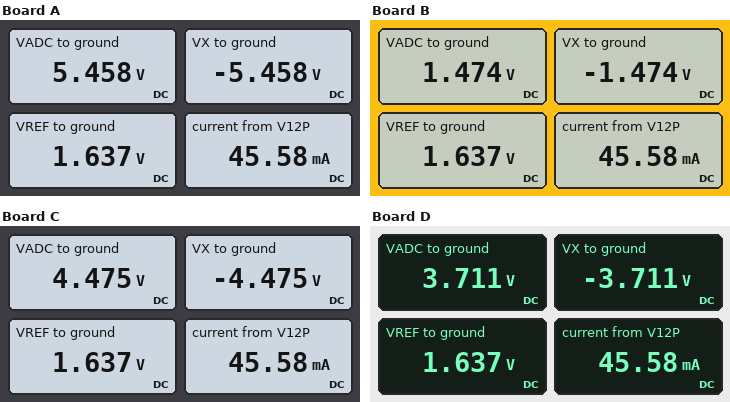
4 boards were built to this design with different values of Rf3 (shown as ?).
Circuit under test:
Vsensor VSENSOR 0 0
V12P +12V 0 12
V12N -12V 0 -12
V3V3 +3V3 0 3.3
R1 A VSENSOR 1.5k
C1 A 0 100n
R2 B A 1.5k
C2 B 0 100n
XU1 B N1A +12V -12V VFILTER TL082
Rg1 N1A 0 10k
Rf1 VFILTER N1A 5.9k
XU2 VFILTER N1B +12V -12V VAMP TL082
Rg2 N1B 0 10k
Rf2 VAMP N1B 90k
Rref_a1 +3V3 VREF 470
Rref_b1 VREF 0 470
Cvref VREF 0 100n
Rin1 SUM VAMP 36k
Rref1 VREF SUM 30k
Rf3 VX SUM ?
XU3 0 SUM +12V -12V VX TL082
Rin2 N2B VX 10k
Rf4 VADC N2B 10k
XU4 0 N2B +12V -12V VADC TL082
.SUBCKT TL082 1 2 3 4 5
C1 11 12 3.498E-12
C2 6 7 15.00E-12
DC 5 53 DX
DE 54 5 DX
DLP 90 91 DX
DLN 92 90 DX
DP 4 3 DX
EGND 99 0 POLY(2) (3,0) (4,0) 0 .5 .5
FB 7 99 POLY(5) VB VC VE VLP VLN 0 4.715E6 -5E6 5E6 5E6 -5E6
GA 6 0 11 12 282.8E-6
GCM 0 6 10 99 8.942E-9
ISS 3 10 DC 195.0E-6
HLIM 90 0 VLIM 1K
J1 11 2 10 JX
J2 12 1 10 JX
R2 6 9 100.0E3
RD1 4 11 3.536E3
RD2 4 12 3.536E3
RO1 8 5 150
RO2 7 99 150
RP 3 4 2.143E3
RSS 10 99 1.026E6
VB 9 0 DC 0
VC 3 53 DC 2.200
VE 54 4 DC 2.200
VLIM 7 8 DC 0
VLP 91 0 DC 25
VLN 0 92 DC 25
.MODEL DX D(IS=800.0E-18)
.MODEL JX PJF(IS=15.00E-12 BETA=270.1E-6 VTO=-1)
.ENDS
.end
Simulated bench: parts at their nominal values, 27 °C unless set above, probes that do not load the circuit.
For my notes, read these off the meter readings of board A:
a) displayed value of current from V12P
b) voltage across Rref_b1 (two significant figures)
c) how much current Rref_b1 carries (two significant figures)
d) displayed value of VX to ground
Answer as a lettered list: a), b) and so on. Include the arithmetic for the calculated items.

a) 45.58 mA
b) 1.637 V = 1.6 V
c) (1.637 V) / 470 Ω = 3.5 mA
d) -5.458 V
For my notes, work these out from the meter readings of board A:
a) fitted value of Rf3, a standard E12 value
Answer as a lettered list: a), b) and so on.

a) 100 kΩ
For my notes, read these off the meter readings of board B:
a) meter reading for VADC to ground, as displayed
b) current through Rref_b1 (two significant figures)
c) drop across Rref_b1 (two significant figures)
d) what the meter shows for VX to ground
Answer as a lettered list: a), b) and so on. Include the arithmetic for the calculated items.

a) 1.474 V
b) (1.637 V) / 470 Ω = 3.5 mA
c) 1.637 V = 1.6 V
d) -1.474 V
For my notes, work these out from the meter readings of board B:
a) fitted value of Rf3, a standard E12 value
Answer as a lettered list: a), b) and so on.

a) 27 kΩ
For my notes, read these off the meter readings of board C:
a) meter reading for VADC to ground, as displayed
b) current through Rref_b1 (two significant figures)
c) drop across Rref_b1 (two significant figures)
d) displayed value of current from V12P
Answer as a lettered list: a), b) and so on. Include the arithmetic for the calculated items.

a) 4.475 V
b) (1.637 V) / 470 Ω = 3.5 mA
c) 1.637 V = 1.6 V
d) 45.58 mA
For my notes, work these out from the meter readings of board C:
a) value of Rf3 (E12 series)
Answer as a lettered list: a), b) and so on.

a) 82 kΩ
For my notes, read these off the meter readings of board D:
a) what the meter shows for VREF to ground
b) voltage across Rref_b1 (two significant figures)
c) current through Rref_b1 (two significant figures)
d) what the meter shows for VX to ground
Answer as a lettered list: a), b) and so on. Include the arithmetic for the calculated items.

a) 1.637 V
b) 1.637 V = 1.6 V
c) (1.637 V) / 470 Ω = 3.5 mA
d) -3.711 V
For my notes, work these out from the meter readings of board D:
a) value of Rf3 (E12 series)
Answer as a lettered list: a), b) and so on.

a) 68 kΩ
